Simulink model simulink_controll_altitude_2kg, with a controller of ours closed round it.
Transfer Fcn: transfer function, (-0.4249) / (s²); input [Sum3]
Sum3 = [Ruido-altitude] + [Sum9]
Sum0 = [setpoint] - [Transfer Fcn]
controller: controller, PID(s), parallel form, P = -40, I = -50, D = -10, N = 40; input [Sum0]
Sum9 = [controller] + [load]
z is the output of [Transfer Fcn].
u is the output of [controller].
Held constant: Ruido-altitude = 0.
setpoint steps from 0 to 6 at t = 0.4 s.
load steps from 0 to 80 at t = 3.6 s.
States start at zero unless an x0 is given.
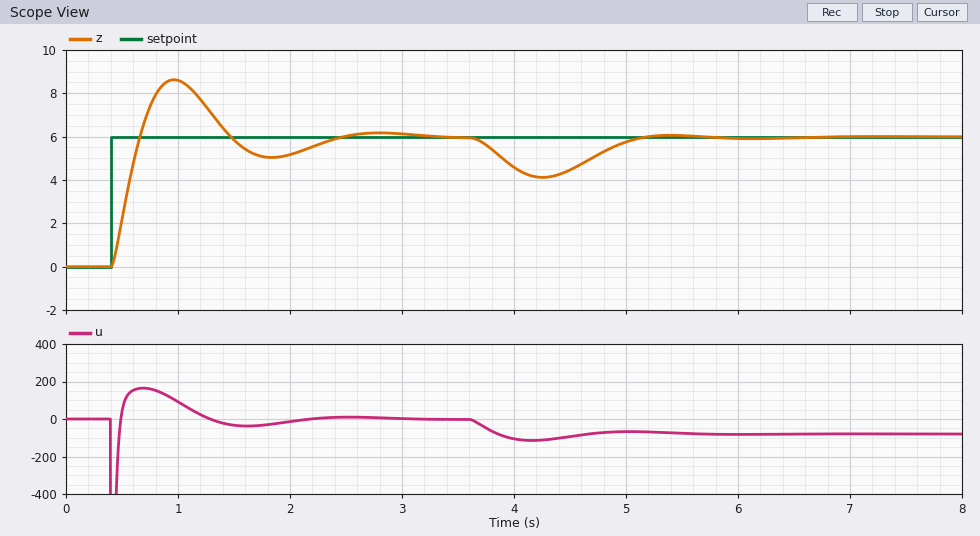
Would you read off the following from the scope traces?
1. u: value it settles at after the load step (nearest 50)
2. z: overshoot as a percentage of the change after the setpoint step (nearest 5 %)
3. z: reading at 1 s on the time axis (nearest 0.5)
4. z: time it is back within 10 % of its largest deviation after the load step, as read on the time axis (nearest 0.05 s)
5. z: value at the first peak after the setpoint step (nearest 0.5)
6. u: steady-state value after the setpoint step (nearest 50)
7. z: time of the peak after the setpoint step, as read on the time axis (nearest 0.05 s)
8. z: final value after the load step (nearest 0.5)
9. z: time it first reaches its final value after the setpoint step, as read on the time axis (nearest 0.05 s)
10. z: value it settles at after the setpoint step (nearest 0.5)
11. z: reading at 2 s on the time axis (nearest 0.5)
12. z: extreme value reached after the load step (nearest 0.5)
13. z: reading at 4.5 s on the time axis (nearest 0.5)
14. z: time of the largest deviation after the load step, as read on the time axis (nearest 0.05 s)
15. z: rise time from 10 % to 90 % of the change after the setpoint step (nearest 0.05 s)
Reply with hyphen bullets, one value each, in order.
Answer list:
- -100
- 45 %
- 8.5
- 5.05 s
- 8.5
- 0
- 0.95 s
- 6.0
- 0.65 s
- 6.0
- 5.0
- 4.0
- 4.5
- 4.25 s
- 0.20 s
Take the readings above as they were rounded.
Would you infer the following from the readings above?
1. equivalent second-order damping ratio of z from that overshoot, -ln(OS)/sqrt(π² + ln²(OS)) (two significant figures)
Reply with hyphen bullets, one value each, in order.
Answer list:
- 0.25
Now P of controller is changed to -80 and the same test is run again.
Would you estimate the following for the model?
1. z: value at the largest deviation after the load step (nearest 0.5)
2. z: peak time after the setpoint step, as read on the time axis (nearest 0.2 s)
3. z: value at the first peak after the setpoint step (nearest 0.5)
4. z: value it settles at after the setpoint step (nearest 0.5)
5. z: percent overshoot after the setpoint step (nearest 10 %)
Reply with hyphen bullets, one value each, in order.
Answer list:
- 5.0
- 0.8 s
- 9.0
- 6.0
- 50 %
